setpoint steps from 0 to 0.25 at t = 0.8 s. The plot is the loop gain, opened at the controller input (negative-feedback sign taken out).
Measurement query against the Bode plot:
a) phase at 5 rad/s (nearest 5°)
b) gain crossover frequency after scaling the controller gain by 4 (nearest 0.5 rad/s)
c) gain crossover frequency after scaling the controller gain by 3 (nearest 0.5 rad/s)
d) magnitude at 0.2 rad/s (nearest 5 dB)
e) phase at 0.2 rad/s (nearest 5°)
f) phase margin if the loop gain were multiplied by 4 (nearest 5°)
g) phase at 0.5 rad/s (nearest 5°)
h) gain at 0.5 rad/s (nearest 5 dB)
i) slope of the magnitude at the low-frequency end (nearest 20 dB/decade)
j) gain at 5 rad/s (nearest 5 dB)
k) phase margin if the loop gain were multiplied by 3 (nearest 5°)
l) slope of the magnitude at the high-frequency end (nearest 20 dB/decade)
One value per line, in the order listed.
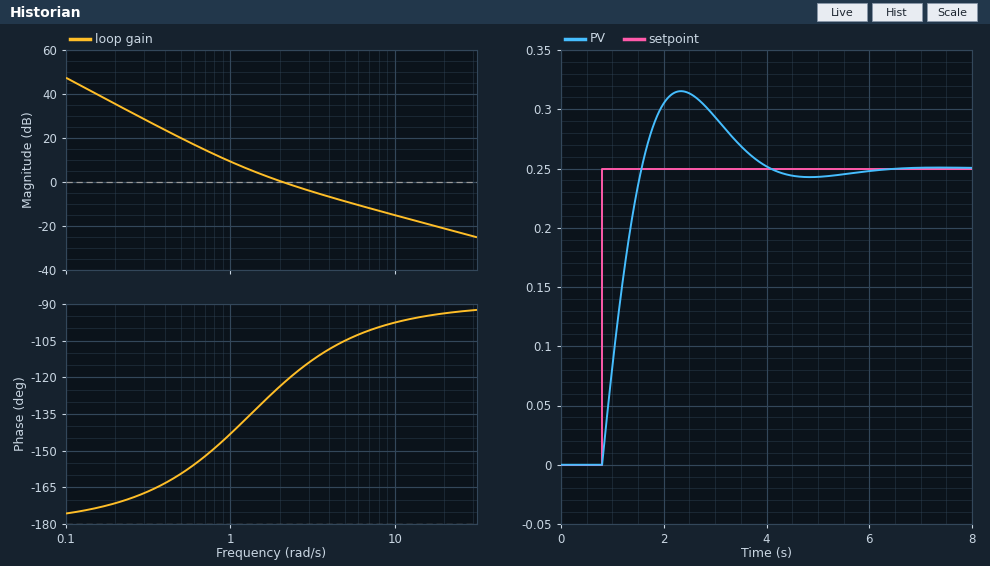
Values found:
-105°
7.0 rad/s
5.5 rad/s
35 dB
-170°
80°
-160°
20 dB
-40 dB/decade
-10 dB
75°
-20 dB/decade
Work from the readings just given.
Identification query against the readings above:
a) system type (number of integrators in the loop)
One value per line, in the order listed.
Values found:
2
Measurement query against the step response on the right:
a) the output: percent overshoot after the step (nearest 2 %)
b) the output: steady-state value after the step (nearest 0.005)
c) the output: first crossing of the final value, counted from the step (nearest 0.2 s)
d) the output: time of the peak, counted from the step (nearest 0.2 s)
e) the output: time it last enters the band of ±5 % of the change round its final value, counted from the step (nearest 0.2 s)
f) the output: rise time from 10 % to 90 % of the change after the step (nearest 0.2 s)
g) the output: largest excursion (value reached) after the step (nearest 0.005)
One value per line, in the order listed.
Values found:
26 %
0.250
0.8 s
1.6 s
2.8 s
0.6 s
0.315
